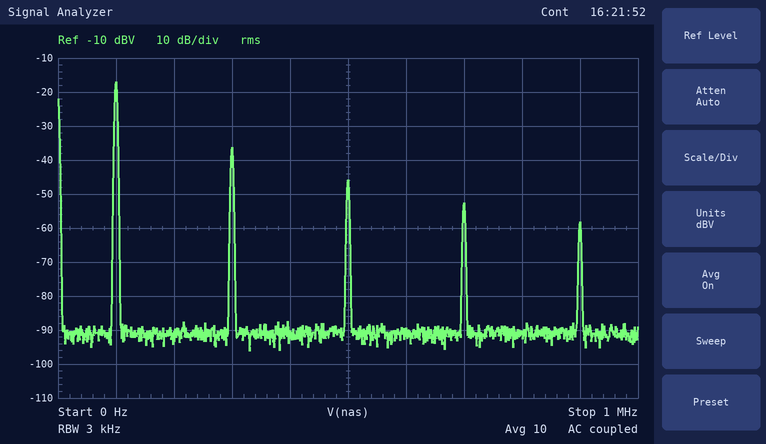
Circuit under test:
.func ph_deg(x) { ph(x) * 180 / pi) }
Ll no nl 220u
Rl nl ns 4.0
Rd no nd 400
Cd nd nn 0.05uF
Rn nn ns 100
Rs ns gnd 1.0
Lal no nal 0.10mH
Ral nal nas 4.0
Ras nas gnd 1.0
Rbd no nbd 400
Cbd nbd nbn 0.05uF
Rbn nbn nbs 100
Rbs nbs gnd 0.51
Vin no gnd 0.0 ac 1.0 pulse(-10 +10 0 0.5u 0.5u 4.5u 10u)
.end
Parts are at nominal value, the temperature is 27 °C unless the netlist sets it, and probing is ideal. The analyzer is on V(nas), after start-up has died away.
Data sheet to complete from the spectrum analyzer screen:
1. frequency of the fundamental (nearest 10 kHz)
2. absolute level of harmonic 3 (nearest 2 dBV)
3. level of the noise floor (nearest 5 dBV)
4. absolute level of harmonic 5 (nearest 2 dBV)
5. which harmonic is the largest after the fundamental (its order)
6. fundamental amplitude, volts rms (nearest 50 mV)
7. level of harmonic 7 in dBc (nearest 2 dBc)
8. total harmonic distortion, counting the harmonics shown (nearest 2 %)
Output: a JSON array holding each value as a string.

["100 kHz", "-36 dBV", "-90 dBV", "-46 dBV", "3", "150 mV", "-36 dBc", "12 %"]
